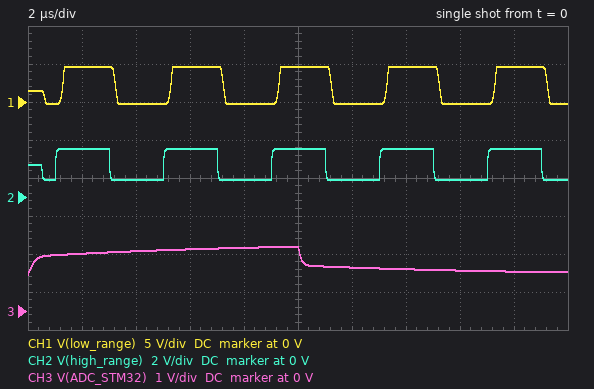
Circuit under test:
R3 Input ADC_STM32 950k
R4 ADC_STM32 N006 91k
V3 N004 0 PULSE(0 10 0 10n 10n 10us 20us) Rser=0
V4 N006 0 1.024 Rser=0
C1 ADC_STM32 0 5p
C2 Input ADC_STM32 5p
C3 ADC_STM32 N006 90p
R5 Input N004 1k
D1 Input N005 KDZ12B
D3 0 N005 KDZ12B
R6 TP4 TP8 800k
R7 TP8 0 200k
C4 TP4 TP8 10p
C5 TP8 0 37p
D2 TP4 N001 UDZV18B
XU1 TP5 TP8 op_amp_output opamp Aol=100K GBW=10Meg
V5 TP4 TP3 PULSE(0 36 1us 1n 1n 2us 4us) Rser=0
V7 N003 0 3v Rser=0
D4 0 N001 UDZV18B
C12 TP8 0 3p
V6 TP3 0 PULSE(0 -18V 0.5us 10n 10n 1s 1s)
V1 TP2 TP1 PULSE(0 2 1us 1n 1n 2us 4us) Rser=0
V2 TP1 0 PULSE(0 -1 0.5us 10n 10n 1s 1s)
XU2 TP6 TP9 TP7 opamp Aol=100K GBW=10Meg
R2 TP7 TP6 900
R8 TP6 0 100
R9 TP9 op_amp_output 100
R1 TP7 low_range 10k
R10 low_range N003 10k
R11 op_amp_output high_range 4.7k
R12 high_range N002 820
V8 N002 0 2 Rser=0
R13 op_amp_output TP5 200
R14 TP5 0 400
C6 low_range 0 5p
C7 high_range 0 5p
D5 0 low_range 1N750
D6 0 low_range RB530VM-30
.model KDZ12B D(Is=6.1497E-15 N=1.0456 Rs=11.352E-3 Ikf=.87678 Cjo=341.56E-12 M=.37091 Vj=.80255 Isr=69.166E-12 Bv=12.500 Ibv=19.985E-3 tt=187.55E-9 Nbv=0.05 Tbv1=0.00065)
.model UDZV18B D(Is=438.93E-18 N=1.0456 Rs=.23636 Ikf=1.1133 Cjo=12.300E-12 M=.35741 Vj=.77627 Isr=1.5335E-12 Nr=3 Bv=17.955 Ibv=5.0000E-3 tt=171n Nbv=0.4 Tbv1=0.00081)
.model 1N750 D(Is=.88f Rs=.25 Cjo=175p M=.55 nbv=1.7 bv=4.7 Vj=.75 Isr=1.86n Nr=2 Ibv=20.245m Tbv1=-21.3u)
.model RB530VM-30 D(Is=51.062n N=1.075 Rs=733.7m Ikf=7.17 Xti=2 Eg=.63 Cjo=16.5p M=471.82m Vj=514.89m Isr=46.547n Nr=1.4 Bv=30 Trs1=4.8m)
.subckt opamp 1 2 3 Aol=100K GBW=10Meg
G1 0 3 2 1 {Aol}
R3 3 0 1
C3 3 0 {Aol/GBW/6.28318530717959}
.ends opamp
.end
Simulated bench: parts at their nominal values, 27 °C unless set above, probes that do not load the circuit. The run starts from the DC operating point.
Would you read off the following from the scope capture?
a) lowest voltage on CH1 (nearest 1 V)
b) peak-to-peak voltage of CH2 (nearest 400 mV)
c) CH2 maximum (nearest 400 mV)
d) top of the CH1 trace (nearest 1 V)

0 V
1.6 V
2.4 V
5 V
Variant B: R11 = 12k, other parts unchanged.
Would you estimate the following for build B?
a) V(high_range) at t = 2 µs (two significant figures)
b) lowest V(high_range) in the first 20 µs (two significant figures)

2.2 V
1.5 V
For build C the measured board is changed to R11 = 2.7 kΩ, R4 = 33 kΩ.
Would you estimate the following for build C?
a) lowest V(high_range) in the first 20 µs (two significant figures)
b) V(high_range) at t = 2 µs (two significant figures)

280 mV
2.8 V
